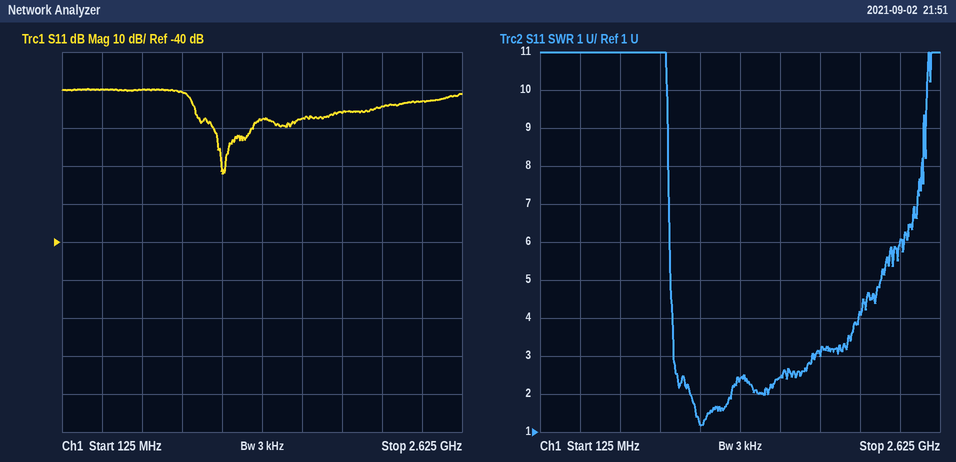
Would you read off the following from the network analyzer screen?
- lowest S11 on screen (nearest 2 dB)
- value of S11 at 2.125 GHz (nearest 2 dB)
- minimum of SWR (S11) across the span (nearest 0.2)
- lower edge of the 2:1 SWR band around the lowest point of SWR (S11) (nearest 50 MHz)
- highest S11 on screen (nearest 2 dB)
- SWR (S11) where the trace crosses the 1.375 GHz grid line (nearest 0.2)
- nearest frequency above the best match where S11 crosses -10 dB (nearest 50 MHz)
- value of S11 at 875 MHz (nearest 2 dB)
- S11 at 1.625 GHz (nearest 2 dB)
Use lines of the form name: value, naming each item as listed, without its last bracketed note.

lowest S11 on screen: -22 dB
value of S11 at 2.125 GHz: -4 dB
minimum of SWR (S11) across the span: 1.2
lower edge of the 2:1 SWR band around the lowest point of SWR (S11): 1.05 GHz
highest S11 on screen: 0 dB
SWR (S11) where the trace crosses the 1.375 GHz grid line: 2.4
nearest frequency above the best match where S11 crosses -10 dB: 1.30 GHz
value of S11 at 875 MHz: 0 dB
S11 at 1.625 GHz: -8 dB
